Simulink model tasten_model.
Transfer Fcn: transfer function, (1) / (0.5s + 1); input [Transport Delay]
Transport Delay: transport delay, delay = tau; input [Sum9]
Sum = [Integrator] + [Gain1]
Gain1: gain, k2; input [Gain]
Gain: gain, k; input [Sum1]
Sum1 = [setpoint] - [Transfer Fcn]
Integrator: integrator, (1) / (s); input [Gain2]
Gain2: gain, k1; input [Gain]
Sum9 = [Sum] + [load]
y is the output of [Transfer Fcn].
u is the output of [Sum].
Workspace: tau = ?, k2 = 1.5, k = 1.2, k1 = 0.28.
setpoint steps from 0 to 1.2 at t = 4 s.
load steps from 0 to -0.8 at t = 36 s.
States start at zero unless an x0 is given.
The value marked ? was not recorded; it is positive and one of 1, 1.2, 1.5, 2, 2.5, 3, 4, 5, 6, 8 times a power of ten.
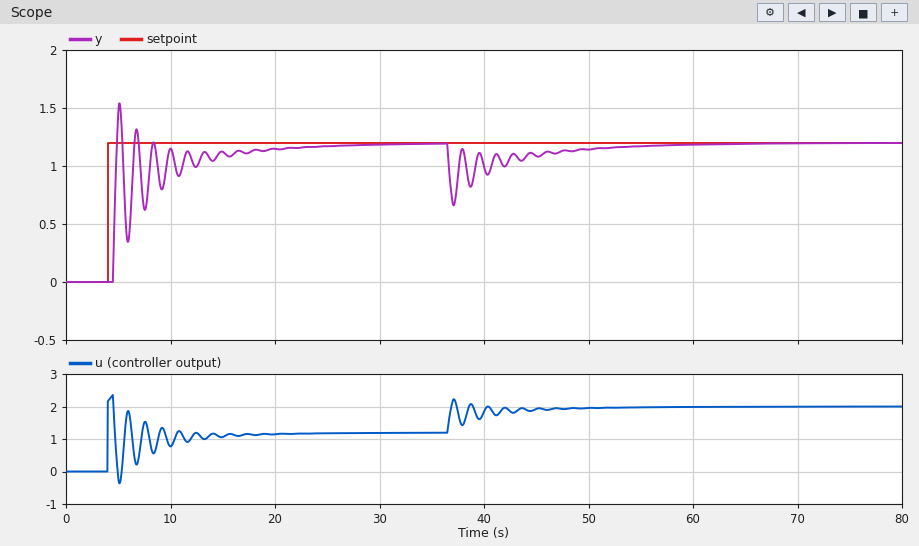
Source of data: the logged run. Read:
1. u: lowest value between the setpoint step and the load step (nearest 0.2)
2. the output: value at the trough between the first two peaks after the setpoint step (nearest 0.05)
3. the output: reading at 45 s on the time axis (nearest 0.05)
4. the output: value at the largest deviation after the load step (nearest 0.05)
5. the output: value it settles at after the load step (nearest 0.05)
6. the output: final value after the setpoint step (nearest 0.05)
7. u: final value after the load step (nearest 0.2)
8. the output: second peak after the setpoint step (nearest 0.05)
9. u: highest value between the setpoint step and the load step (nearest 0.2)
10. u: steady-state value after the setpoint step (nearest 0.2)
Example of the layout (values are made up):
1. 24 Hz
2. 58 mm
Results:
1. -0.4
2. 0.35
3. 1.10
4. 0.65
5. 1.20
6. 1.20
7. 2.0
8. 1.30
9. 2.4
10. 1.2
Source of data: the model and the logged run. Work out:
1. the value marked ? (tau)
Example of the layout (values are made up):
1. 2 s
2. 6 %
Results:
1. 0.5
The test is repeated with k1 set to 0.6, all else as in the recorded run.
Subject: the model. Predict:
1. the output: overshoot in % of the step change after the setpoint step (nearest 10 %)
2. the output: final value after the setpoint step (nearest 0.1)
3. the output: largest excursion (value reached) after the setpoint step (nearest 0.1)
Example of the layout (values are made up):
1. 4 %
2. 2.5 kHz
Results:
1. 40 %
2. 1.2
3. 1.7
